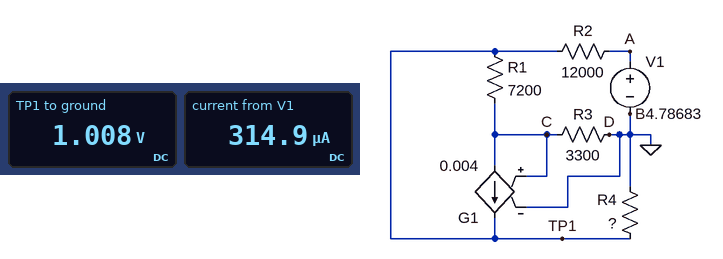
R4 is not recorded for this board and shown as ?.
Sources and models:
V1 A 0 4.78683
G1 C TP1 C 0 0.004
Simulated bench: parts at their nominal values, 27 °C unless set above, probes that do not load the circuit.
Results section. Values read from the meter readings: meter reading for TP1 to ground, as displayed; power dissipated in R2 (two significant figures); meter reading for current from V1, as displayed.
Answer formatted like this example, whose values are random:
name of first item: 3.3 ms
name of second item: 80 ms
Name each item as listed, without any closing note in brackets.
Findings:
meter reading for TP1 to ground, as displayed: 1.008 V
power dissipated in R2: 1.2 mW
meter reading for current from V1, as displayed: 314.9 µA
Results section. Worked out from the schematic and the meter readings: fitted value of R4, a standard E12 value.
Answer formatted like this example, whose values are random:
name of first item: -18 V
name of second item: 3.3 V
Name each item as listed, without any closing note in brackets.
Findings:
fitted value of R4, a standard E12 value: 3.3 kΩ
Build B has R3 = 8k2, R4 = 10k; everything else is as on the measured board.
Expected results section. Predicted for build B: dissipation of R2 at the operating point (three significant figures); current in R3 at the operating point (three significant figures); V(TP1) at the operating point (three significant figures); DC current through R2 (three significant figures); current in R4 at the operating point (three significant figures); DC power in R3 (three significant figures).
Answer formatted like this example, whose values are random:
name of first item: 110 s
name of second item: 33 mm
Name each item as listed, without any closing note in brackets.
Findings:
dissipation of R2 at the operating point: 588 µW
current in R3 at the operating point: 8.47 µA
V(TP1) at the operating point: 2.13 V
DC current through R2: 221 µA
current in R4 at the operating point: 213 µA
DC power in R3: 588 nW
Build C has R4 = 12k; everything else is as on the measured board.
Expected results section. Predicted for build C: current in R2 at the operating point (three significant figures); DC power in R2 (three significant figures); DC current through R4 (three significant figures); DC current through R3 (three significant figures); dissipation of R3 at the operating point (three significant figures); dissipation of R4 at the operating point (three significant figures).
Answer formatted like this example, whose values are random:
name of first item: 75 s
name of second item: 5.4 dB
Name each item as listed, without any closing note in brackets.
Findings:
current in R2 at the operating point: 210 µA
DC power in R2: 530 µW
DC current through R4: 189 µA
DC current through R3: 21.5 µA
dissipation of R3 at the operating point: 1.52 µW
dissipation of R4 at the operating point: 427 µW
